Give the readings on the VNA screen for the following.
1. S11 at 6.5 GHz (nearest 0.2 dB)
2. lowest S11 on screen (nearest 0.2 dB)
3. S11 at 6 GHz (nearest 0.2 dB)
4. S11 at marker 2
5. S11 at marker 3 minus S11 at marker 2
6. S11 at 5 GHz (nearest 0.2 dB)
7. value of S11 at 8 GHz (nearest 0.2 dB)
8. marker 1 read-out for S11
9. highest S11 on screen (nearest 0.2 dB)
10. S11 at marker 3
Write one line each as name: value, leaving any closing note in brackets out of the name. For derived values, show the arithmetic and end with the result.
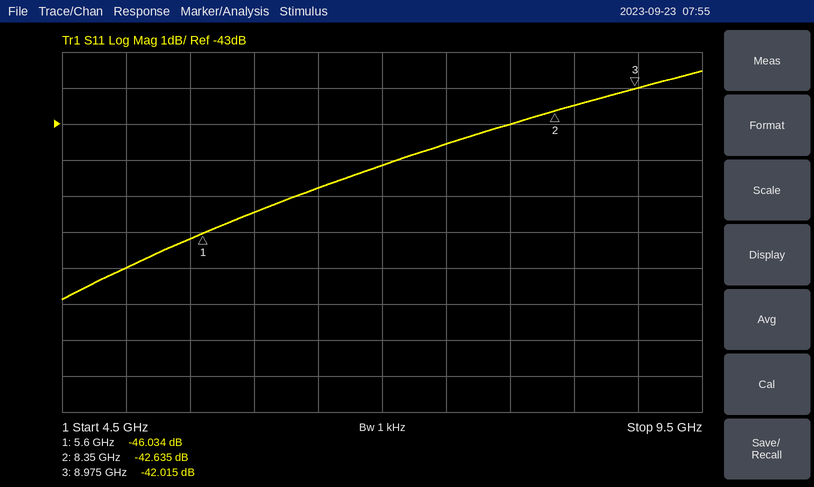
S11 at 6.5 GHz: -44.8 dB
lowest S11 on screen: -47.8 dB
S11 at 6 GHz: -45.4 dB
S11 at marker 2: -42.635 dB
S11 at marker 3 minus S11 at marker 2: -42.015 − (-42.635) = 0.620 dB
S11 at 5 GHz: -47.0 dB
value of S11 at 8 GHz: -43.0 dB
marker 1 read-out for S11: -46.034 dB
highest S11 on screen: -41.6 dB
S11 at marker 3: -42.015 dB
